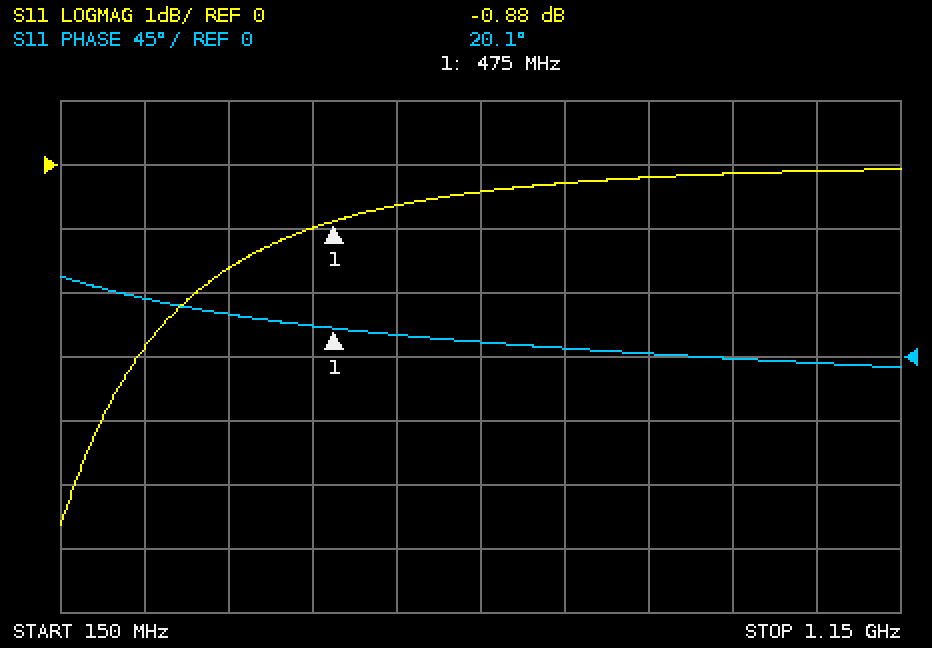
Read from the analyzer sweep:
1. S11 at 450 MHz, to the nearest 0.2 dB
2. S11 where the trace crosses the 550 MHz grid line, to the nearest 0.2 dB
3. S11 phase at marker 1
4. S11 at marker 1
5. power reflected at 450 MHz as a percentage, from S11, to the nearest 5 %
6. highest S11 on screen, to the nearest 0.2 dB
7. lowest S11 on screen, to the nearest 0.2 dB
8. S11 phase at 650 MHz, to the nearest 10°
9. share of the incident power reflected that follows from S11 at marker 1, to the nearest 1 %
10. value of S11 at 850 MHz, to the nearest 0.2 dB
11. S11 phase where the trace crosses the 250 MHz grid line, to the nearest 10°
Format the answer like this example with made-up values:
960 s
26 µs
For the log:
-1.0 dB
-0.6 dB
20.1°
-0.88 dB
80 %
0.0 dB
-5.6 dB
10°
82 %
-0.2 dB
40°
